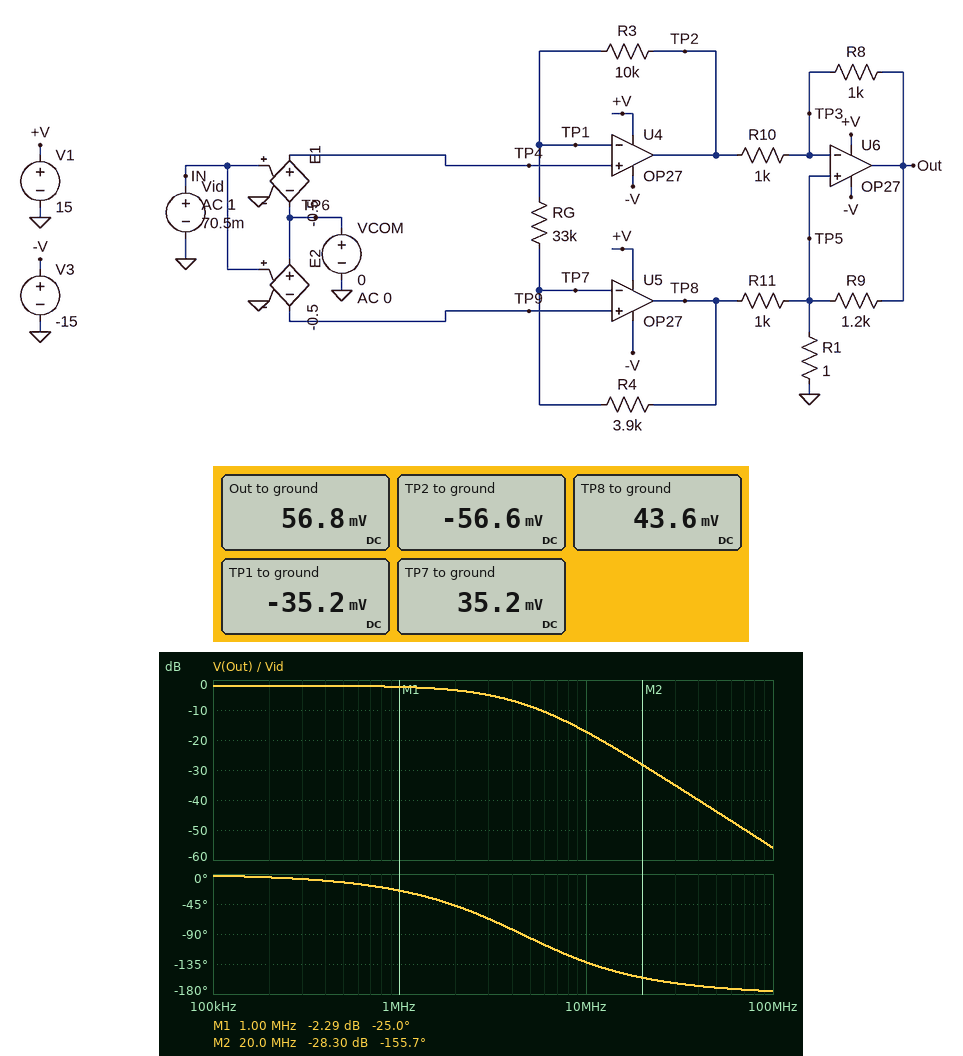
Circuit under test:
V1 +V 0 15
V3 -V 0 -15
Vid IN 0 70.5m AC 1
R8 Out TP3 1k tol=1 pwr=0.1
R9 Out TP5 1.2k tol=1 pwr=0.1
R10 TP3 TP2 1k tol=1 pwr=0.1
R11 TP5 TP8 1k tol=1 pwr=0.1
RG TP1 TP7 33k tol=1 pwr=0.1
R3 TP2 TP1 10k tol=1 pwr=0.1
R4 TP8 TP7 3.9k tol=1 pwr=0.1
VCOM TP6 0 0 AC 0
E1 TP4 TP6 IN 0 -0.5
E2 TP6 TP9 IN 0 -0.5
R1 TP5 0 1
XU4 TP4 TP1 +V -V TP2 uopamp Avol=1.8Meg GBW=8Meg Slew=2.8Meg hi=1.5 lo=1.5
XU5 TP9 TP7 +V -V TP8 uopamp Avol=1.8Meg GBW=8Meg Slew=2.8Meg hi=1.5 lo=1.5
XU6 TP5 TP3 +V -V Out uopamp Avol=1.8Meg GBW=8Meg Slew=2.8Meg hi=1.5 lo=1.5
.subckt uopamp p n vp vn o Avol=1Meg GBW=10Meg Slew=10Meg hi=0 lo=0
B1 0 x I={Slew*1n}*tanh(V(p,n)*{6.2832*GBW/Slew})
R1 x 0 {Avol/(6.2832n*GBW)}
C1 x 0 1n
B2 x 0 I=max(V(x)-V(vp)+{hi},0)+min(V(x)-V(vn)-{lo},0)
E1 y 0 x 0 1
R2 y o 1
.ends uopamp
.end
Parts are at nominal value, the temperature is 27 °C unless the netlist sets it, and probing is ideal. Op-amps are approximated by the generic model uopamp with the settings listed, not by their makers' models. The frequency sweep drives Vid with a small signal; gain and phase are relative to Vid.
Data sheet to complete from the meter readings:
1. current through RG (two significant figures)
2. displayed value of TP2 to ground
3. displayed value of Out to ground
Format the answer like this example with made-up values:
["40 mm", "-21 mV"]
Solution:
["2.1 µA", "-56.6 mV", "56.8 mV"]
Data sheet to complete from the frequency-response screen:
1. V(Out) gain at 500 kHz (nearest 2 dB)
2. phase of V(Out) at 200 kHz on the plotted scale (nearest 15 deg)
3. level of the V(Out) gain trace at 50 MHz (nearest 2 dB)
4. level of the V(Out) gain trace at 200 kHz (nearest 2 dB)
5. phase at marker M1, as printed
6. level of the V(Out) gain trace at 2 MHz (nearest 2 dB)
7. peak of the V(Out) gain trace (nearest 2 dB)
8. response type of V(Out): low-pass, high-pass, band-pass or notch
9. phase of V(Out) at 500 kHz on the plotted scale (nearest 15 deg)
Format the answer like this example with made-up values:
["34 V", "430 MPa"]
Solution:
["-2 dB", "0 deg", "-44 dB", "-2 dB", "-25.0 deg", "-4 dB", "-2 dB", "low-pass", "-15 deg"]
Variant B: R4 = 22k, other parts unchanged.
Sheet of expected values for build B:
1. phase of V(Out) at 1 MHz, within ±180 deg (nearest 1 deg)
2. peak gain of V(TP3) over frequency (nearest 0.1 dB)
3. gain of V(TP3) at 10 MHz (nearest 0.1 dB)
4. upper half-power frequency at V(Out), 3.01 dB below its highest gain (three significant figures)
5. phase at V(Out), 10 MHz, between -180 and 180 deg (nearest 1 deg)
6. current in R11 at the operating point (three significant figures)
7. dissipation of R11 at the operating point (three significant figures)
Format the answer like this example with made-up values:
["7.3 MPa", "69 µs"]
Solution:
["-26 deg", "-13.4 dB", "-15.9 dB", "2.70 MHz", "-131 deg", "82.1 µA", "6.74 µW"]
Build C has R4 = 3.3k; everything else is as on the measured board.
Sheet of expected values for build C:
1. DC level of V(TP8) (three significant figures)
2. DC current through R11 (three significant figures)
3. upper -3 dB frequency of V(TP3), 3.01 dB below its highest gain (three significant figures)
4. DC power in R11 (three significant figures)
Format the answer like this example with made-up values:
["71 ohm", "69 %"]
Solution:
["42.3 mV", "42.2 µA", "10.8 MHz", "1.78 µW"]
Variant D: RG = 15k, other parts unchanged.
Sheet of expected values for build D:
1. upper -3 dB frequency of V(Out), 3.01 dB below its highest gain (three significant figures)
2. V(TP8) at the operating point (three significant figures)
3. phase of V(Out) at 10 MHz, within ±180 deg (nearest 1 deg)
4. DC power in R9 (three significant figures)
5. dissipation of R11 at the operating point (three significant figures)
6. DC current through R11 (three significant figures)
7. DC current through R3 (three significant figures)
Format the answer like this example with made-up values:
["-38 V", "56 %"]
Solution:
["2.55 MHz", "53.6 mV", "-141 deg", "5.65 µW", "2.86 µW", "53.5 µA", "4.70 µA"]
